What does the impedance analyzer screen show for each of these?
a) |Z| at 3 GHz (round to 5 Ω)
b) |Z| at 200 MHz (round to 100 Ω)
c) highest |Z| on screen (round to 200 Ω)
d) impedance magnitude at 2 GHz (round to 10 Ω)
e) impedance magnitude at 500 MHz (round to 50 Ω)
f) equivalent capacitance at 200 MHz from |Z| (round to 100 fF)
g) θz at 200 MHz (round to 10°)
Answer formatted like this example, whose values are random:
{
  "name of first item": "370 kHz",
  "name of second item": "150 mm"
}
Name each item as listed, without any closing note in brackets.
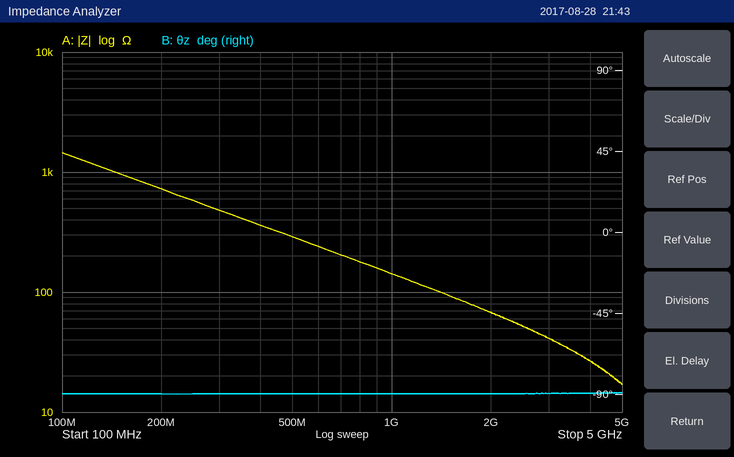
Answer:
{
  "|Z| at 3 GHz": "40 Ω",
  "|Z| at 200 MHz": "700 Ω",
  "highest |Z| on screen": "1.4 kΩ",
  "impedance magnitude at 2 GHz": "70 Ω",
  "impedance magnitude at 500 MHz": "300 Ω",
  "equivalent capacitance at 200 MHz from |Z|": "1.1 pF",
  "θz at 200 MHz": "-90°"
}
